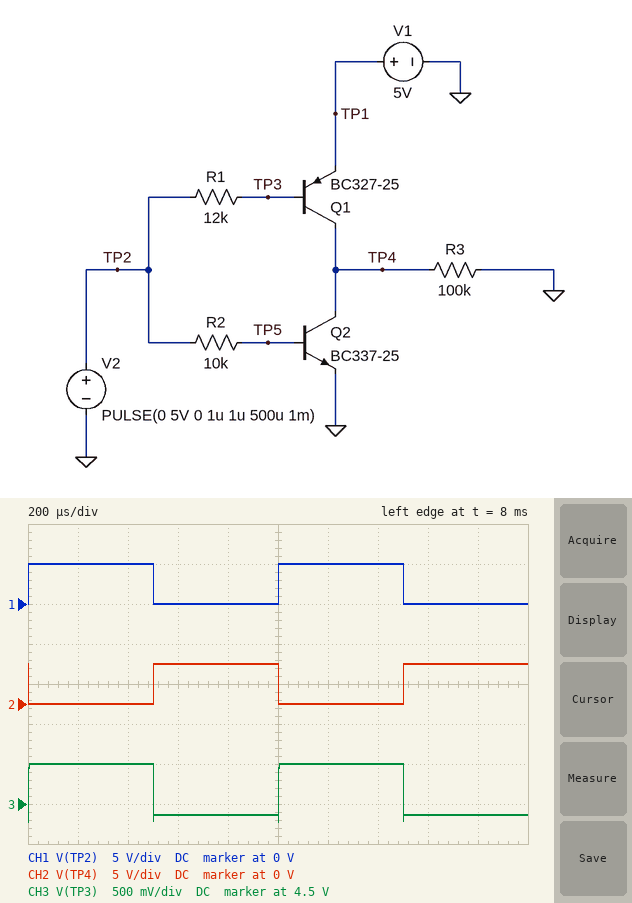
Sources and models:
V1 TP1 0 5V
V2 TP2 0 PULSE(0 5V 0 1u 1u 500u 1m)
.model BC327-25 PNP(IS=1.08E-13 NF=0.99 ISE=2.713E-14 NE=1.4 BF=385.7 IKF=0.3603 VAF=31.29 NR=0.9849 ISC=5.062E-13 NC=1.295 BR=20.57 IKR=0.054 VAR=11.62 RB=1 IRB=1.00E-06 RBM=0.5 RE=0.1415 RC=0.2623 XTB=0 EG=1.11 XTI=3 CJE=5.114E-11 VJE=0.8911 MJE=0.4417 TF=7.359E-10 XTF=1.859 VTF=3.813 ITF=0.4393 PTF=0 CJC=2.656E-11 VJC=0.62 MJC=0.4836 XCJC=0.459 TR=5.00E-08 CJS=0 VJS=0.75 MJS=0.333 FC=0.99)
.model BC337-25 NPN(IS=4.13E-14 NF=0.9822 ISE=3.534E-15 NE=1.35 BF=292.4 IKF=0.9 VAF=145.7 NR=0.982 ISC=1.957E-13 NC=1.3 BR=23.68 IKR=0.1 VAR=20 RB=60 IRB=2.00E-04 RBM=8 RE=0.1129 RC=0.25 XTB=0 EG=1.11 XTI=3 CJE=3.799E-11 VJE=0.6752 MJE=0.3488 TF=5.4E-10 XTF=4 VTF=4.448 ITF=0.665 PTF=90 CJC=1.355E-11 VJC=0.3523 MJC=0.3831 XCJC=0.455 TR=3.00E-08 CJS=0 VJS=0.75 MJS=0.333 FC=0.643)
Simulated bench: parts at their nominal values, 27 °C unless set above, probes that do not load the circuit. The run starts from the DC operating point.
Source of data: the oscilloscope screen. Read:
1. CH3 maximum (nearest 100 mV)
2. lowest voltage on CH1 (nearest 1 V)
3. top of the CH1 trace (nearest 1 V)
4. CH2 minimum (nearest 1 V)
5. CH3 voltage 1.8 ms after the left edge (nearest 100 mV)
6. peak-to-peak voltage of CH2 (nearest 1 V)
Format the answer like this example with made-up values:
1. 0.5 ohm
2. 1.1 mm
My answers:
1. 5.0 V
2. 0 V
3. 5 V
4. 0 V
5. 4.4 V
6. 5 V
